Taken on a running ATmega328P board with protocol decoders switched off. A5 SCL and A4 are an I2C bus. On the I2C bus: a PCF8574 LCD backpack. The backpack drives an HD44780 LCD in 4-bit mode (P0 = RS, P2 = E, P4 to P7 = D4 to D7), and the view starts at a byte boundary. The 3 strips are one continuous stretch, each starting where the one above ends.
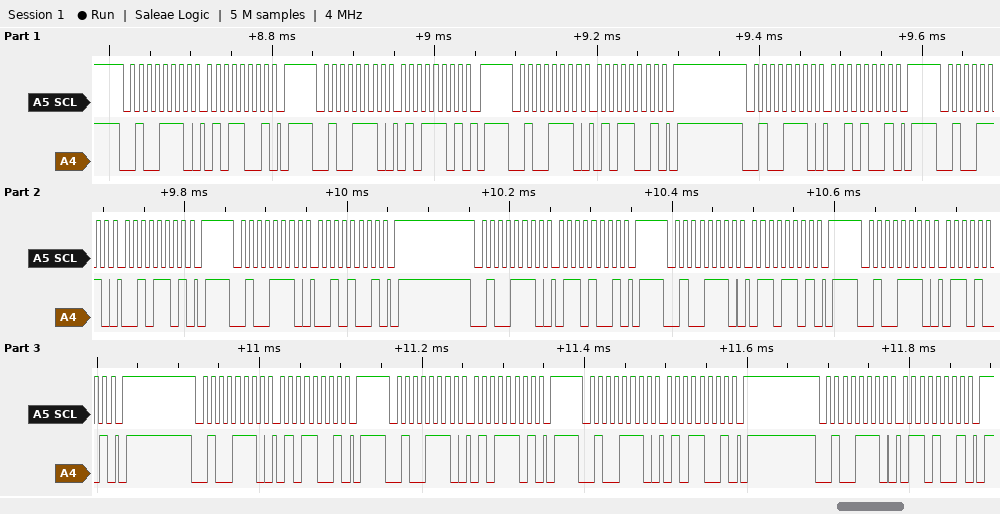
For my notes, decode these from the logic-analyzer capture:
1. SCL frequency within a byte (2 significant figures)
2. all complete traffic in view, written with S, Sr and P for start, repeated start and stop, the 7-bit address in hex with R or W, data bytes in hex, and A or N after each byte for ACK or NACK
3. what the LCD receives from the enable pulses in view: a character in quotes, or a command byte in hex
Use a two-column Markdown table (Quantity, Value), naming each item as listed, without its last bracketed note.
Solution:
| Quantity | Value |
|---|---|
| SCL frequency within a byte | 100 kHz |
| all complete traffic in view, written with S, Sr and P for start, repeated start and stop, the 7-bit address in hex with R or W, data bytes in hex, and A or N after each byte for ACK or NACK | S 27W A 59 A P S 27W A 5D A P S 27W A 59 A P S 27W A 29 A P S 27W A 2D A P S 27W A 29 A P S 27W A 69 A P S 27W A 6D A P S 27W A 69 A P S 27W A 59 A P S 27W A 5D A P S 27W A 59 A P S 27W A 69 A P |
| what the LCD receives from the enable pulses in view: a character in quotes, or a command byte in hex | 'R' 'e' |
